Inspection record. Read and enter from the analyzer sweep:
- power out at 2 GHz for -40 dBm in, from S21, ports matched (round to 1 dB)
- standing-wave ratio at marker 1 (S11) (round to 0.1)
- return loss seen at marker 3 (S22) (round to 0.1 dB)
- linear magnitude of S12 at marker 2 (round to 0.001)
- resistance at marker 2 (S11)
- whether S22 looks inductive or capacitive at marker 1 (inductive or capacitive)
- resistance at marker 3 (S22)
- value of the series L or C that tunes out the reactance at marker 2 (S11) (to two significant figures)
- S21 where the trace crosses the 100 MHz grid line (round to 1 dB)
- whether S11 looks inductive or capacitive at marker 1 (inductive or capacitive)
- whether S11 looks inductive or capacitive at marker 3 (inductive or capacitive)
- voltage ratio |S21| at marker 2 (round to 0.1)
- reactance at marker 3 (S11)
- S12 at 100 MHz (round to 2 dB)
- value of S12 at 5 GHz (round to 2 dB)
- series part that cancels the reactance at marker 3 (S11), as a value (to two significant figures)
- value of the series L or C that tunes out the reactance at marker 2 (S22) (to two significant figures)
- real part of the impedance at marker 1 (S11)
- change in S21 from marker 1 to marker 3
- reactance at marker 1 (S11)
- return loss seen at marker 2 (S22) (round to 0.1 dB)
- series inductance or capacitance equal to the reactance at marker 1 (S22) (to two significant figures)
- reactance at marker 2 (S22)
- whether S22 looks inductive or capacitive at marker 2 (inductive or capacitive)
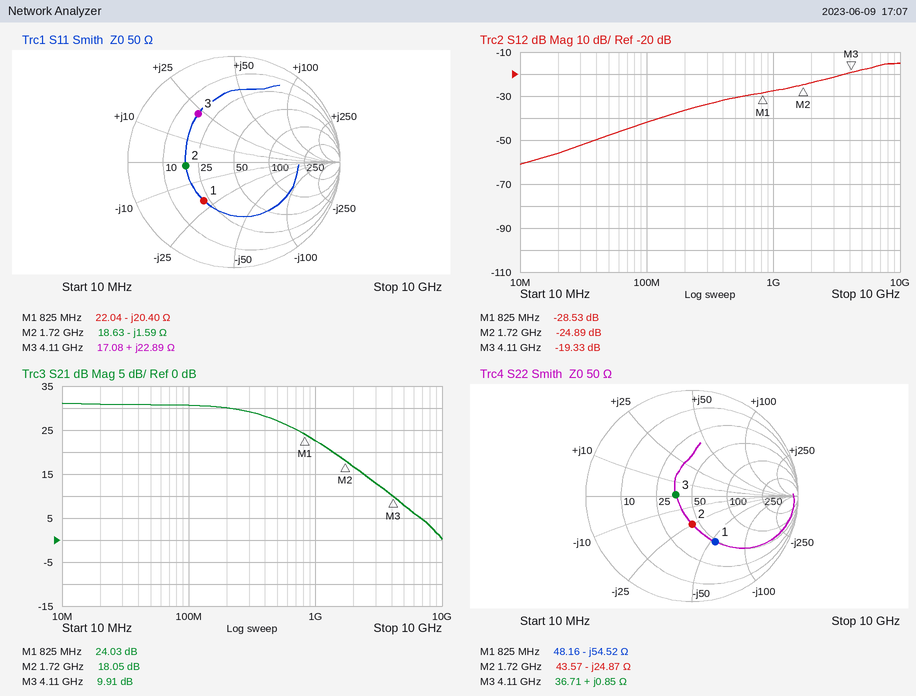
-23 dBm
2.7
16.3 dB
0.057
18.63 Ω
capacitive
36.71 Ω
150 pH
31 dB
capacitive
inductive
8.0
+22.89 Ω
-42 dB
-18 dB
1.7 pF
2.3 nH
22.04 Ω
-14.12 dB
-20.40 Ω
11.5 dB
3.5 pF
-24.87 Ω
capacitive
